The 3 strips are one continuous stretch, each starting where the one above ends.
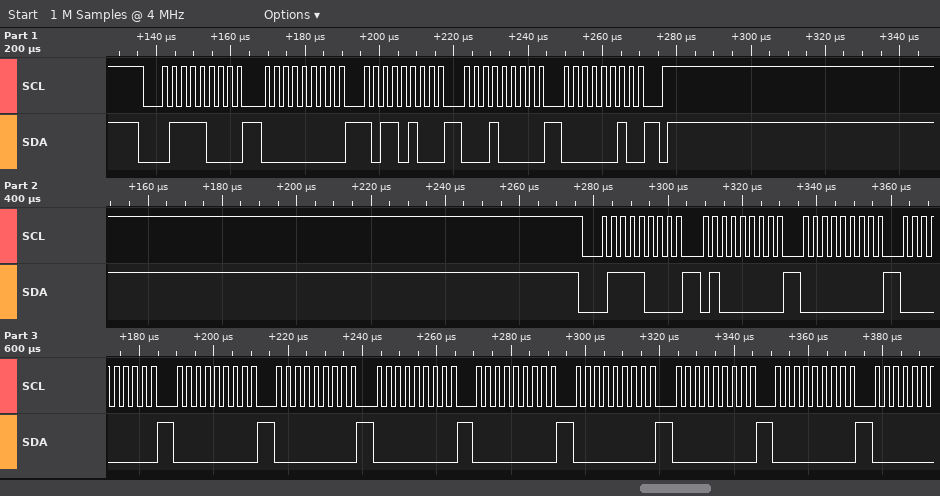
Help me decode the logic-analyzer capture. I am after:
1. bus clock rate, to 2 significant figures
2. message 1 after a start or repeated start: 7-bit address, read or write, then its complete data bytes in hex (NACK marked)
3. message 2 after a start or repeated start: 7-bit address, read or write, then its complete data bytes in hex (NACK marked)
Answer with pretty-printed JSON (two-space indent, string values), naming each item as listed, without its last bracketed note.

{
  "bus clock rate, to 2 significant figures": "400 kHz",
  "message 1 after a start or repeated start: 7-bit address, read or write, then its complete data bytes in hex": "0x3C write: 00 B4 10 02",
  "message 2 after a start or repeated start: 7-bit address, read or write, then its complete data bytes in hex": "0x3C write: 40 00 00 00 00 00 00 00 00 00"
}
